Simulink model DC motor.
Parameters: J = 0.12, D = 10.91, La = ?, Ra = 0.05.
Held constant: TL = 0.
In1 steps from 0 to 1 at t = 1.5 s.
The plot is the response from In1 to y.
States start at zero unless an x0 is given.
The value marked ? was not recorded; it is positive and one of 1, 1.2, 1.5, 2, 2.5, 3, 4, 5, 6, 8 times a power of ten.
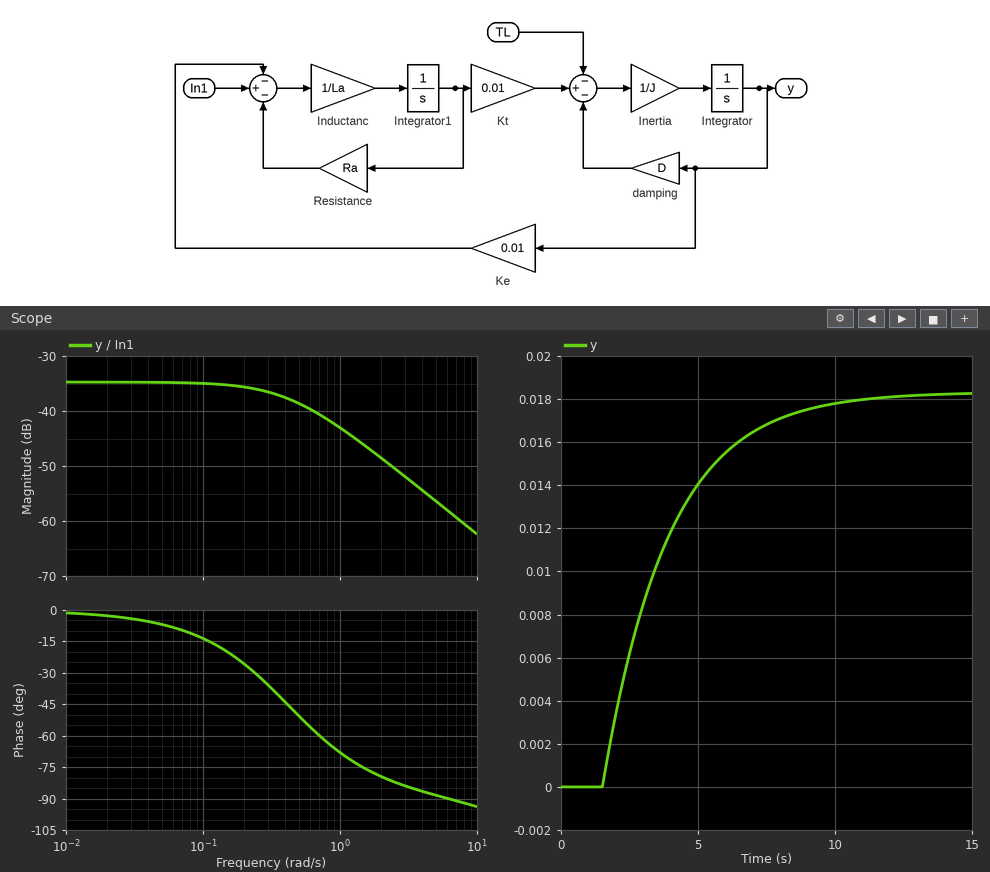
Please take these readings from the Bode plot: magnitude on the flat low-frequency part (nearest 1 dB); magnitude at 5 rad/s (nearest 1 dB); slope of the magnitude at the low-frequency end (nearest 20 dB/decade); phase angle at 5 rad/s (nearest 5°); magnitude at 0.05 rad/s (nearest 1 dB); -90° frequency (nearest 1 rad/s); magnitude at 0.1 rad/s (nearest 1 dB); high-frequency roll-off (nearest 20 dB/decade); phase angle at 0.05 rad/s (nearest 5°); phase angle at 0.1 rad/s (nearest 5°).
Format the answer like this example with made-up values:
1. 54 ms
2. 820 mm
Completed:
1. -35 dB
2. -56 dB
3. 0 dB/decade
4. -90°
5. -35 dB
6. 6 rad/s
7. -35 dB
8. -20 dB/decade
9. -5°
10. -15°
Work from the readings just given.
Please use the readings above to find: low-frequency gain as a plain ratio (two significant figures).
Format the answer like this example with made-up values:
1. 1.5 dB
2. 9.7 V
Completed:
1. 0.018
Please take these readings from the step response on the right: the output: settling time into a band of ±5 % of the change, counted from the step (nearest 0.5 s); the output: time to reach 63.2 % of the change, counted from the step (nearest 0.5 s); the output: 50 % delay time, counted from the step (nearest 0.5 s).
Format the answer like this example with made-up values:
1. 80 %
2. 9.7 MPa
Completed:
1. 7.0 s
2. 2.5 s
3. 1.5 s
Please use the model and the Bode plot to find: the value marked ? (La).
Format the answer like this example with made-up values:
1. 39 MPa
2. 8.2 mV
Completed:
1. 0.12
